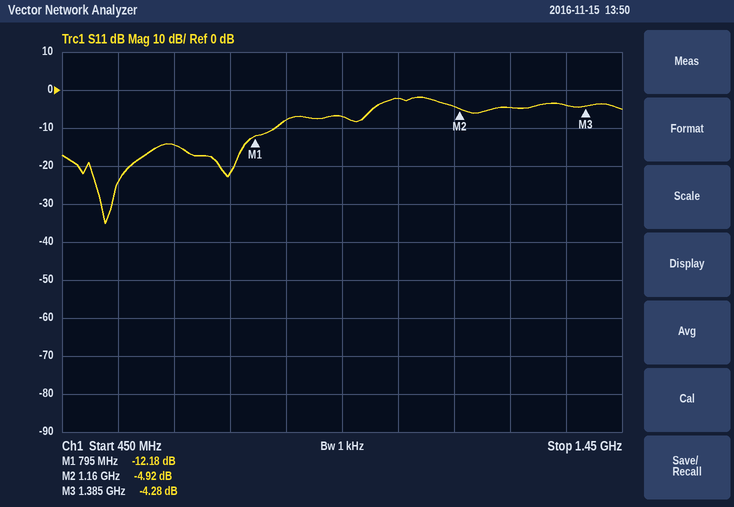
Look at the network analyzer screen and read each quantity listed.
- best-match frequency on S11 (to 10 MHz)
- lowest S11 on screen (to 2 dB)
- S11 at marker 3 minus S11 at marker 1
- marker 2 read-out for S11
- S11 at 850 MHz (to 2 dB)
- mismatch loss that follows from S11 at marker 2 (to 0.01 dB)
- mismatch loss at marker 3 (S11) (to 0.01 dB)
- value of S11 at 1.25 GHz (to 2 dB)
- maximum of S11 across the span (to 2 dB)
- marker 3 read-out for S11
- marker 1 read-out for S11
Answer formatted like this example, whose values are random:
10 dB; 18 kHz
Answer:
530 MHz; -36 dB; 7.90 dB; -4.92 dB; -8 dB; 1.69 dB; 2.03 dB; -4 dB; -2 dB; -4.28 dB; -12.18 dB
